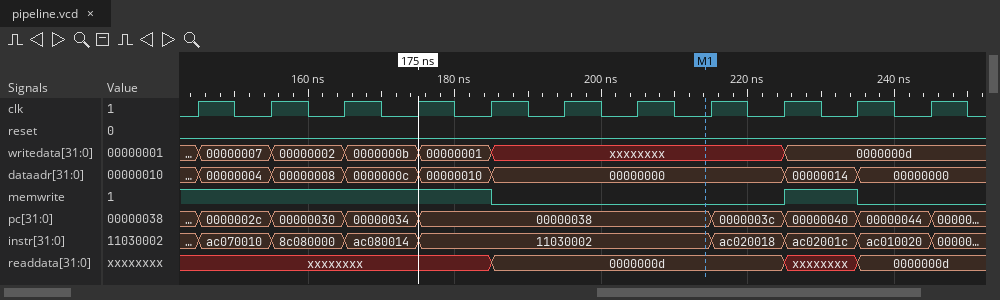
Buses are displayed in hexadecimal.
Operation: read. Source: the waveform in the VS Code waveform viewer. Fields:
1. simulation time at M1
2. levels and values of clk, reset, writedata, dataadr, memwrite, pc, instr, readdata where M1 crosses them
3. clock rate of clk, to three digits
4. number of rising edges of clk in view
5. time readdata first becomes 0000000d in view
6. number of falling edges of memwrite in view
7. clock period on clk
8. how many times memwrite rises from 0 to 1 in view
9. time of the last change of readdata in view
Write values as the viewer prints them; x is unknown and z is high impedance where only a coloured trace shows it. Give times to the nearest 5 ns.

215 ns
clk=0, reset=0, writedata=xxxxxxxx, dataadr=00000000, memwrite=0, pc=00000038, instr=11030002, readdata=0000000d
100 MHz
11
185 ns
2
10 ns
1
235 ns
